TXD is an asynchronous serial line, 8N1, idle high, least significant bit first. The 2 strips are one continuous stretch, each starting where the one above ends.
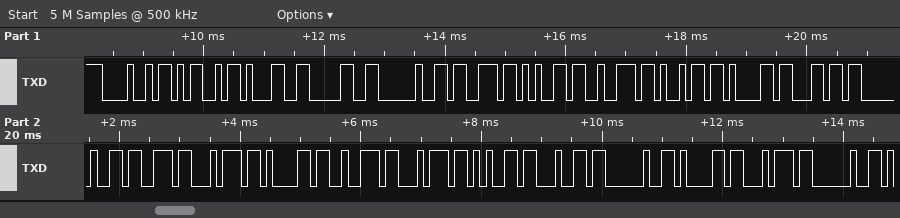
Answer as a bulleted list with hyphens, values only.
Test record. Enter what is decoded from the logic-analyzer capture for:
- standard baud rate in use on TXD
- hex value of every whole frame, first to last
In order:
- 9600 baud
- 48 4D 31 30 20 73 65 72 69 61 6C 20 73 74 61 72 74 65 64 20 61 74 20
